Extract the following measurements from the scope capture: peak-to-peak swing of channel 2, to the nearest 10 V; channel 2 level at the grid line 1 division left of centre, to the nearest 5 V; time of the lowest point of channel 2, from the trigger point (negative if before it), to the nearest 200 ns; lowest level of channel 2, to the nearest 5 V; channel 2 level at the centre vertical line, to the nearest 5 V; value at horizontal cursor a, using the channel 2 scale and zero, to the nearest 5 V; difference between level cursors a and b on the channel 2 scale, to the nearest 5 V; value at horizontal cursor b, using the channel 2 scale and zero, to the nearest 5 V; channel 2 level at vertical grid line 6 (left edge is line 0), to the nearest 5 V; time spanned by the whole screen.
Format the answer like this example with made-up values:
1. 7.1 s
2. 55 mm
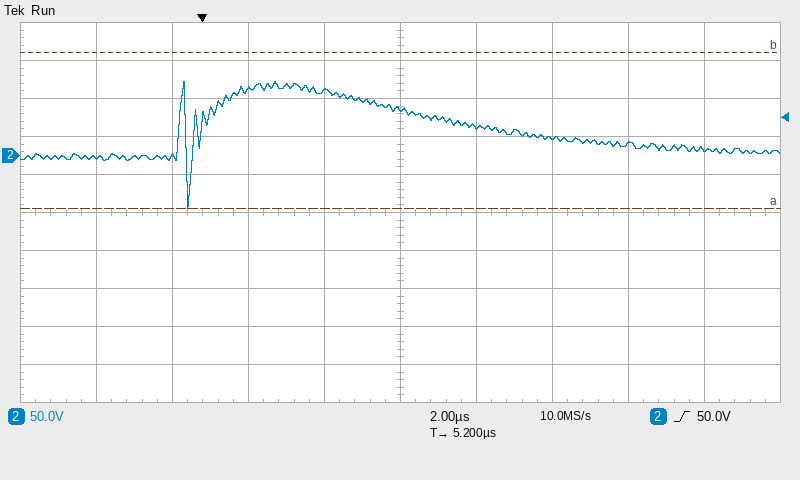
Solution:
1. 170 V
2. 85 V
3. -400 ns
4. -70 V
5. 60 V
6. -70 V
7. 205 V
8. 135 V
9. 40 V
10. 20 µs
